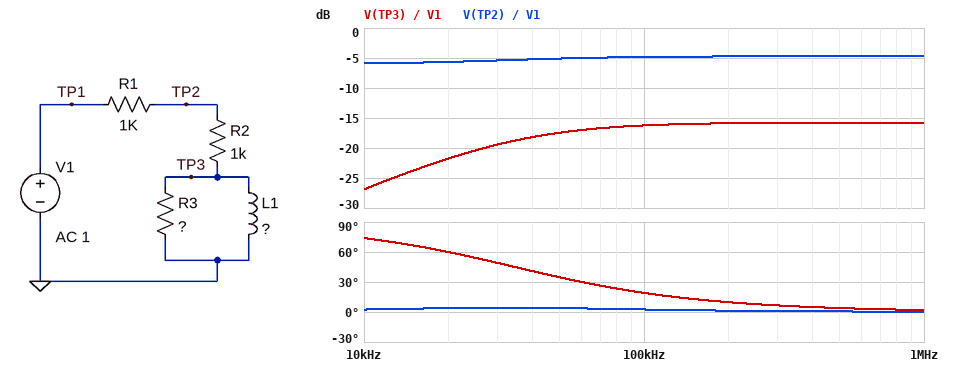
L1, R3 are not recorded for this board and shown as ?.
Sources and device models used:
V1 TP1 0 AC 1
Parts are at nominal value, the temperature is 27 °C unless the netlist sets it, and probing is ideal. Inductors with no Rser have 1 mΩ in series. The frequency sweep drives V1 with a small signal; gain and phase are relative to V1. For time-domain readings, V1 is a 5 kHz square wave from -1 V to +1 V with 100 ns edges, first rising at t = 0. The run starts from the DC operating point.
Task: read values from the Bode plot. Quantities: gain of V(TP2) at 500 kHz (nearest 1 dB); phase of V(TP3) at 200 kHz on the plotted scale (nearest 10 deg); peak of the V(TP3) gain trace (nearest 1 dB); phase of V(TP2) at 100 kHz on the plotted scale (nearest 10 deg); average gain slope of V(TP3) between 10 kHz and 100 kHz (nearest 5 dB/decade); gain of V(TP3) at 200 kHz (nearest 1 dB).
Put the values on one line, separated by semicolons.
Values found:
-5 dB; 10 deg; -16 dB; 0 deg; 10 dB/decade; -16 dB
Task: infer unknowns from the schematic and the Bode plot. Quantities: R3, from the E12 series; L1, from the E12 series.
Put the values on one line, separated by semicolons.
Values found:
390 Ω; 1.5 mH
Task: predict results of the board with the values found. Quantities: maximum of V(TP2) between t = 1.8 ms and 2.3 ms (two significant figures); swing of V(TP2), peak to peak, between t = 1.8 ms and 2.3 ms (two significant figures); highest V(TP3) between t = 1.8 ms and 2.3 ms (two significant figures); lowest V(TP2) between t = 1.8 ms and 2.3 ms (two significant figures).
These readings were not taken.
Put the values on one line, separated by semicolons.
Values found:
660 mV; 1.3 V; 320 mV; -660 mV
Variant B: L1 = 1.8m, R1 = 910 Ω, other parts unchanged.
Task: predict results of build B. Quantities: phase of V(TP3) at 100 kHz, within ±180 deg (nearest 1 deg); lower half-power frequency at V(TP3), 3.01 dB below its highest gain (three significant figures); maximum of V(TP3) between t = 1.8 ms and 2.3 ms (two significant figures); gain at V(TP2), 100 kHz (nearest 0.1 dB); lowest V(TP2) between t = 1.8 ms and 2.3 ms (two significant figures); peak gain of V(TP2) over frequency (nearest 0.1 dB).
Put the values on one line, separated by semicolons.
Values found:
16 deg; 28.6 kHz; 340 mV; -4.5 dB; -680 mV; -4.4 dB
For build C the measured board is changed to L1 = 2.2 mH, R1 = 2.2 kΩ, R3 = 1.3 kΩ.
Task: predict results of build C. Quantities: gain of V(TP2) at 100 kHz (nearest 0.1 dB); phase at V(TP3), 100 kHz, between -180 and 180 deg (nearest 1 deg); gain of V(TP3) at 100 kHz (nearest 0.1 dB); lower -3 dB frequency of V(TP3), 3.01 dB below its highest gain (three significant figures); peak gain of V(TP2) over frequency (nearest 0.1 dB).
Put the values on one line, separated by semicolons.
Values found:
-6.8 dB; 34 deg; -12.4 dB; 66.9 kHz; -5.8 dB
